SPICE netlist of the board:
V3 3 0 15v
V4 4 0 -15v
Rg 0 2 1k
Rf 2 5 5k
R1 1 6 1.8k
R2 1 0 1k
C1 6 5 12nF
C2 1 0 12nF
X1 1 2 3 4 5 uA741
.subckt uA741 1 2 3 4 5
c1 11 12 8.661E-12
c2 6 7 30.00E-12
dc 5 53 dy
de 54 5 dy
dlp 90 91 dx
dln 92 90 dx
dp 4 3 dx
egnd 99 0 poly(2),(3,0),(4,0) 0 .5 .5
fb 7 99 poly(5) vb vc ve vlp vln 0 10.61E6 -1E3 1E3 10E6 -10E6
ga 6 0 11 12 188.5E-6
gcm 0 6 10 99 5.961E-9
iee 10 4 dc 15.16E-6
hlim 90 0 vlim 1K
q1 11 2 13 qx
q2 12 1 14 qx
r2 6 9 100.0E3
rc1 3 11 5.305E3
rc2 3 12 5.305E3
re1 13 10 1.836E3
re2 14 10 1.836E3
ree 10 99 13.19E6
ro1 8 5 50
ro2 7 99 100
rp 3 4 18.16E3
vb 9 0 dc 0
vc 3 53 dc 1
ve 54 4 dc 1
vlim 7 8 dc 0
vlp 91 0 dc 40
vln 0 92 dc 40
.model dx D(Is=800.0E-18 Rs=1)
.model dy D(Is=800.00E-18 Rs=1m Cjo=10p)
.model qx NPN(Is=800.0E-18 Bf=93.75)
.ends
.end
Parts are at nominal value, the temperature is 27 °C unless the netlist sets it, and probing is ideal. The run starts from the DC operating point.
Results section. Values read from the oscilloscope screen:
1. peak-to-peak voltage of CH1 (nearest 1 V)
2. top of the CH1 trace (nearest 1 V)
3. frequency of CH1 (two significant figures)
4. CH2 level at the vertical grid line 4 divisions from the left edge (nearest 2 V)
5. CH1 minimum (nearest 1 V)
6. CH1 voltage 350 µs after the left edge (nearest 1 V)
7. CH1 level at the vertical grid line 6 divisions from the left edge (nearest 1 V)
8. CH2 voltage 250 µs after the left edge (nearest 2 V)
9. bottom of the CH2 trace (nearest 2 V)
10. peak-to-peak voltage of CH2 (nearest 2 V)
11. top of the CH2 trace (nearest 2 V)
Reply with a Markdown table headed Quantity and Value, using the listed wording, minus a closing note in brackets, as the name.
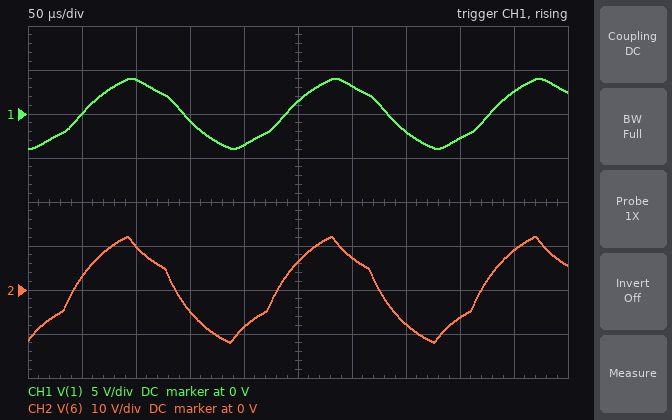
| Quantity | Value |
|---|---|
| peak-to-peak voltage of CH1 | 8 V |
| top of the CH1 trace | 4 V |
| frequency of CH1 | 5.3 kHz |
| CH2 level at the vertical grid line 4 divisions from the left edge | -8 V |
| CH1 minimum | -4 V |
| CH1 voltage 350 µs after the left edge | -2 V |
| CH1 level at the vertical grid line 6 divisions from the left edge | 3 V |
| CH2 voltage 250 µs after the left edge | 6 V |
| bottom of the CH2 trace | -12 V |
| peak-to-peak voltage of CH2 | 24 V |
| top of the CH2 trace | 12 V |
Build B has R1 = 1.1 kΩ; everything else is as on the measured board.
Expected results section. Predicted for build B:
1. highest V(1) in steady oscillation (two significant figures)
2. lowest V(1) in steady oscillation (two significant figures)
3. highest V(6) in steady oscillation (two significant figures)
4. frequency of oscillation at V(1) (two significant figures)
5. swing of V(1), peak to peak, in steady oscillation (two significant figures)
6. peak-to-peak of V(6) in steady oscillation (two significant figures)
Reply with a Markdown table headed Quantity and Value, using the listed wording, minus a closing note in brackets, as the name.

| Quantity | Value |
|---|---|
| highest V(1) in steady oscillation | 4.6 V |
| lowest V(1) in steady oscillation | -4.5 V |
| highest V(6) in steady oscillation | 10 V |
| frequency of oscillation at V(1) | 5.4 kHz |
| swing of V(1), peak to peak, in steady oscillation | 9.1 V |
| peak-to-peak of V(6) in steady oscillation | 20 V |
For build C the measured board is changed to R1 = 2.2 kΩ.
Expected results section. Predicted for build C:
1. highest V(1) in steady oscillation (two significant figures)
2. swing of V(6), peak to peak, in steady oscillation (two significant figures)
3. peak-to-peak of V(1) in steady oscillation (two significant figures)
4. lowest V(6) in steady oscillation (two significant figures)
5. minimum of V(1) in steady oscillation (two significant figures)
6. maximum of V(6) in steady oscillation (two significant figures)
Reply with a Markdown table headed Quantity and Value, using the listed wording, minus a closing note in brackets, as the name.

| Quantity | Value |
|---|---|
| highest V(1) in steady oscillation | 3.7 V |
| swing of V(6), peak to peak, in steady oscillation | 26 V |
| peak-to-peak of V(1) in steady oscillation | 7.4 V |
| lowest V(6) in steady oscillation | -13 V |
| minimum of V(1) in steady oscillation | -3.7 V |
| maximum of V(6) in steady oscillation | 13 V |
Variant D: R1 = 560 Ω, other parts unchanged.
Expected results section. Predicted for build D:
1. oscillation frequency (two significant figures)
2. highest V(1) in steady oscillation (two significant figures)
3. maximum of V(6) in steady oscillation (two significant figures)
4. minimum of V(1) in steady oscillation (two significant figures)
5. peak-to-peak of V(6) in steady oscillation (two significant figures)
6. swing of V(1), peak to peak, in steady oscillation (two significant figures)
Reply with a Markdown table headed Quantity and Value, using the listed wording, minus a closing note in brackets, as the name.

| Quantity | Value |
|---|---|
| oscillation frequency | 5.6 kHz |
| highest V(1) in steady oscillation | 5.0 V |
| maximum of V(6) in steady oscillation | 8.0 V |
| minimum of V(1) in steady oscillation | -4.9 V |
| peak-to-peak of V(6) in steady oscillation | 16 V |
| swing of V(1), peak to peak, in steady oscillation | 9.9 V |
